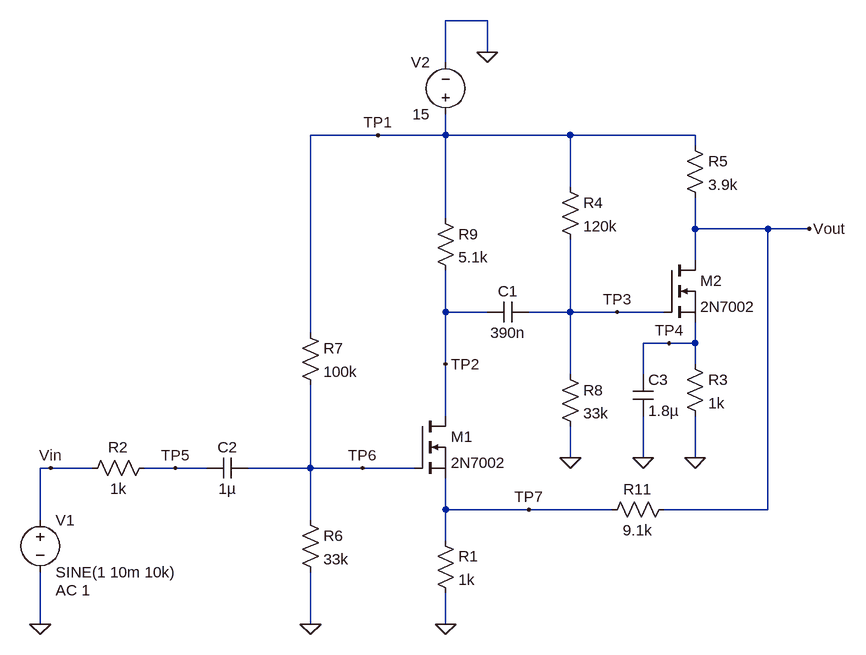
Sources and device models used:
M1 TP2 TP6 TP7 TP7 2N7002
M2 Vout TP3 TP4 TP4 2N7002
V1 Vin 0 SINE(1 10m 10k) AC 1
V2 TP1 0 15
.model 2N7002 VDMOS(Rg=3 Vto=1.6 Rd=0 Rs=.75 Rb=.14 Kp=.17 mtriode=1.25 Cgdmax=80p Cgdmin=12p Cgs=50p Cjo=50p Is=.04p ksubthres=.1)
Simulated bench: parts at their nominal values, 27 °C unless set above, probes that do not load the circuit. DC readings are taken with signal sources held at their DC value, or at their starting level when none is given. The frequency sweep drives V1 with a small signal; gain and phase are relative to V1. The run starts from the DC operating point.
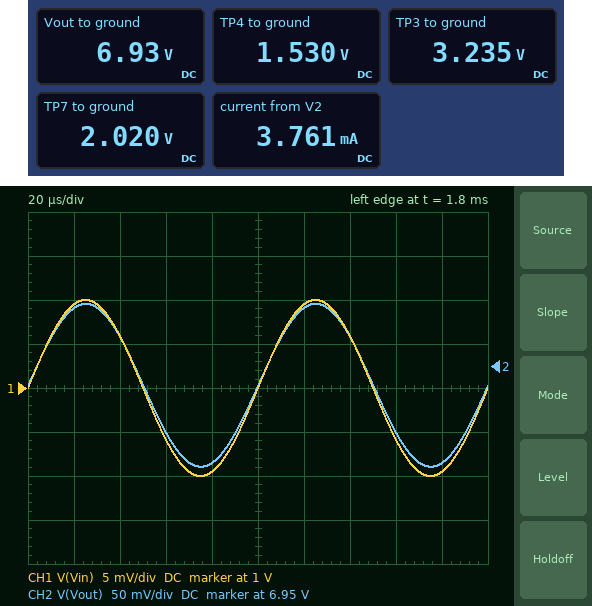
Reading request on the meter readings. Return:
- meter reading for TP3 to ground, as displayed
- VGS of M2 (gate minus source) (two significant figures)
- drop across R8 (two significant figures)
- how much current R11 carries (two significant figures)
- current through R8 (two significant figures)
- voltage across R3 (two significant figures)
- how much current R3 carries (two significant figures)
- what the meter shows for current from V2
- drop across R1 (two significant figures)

3.235 V
1.7 V
3.2 V
540 µA
98 µA
1.5 V
1.5 mA
3.761 mA
2.0 V
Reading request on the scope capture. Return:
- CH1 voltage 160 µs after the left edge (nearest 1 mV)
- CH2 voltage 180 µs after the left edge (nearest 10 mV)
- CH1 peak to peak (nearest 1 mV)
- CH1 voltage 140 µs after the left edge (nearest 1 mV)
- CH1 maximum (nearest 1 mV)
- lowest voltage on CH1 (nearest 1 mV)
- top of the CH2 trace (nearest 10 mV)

994 mV
6.84 V
20 mV
1.006 V
1.010 V
990 mV
7.02 V
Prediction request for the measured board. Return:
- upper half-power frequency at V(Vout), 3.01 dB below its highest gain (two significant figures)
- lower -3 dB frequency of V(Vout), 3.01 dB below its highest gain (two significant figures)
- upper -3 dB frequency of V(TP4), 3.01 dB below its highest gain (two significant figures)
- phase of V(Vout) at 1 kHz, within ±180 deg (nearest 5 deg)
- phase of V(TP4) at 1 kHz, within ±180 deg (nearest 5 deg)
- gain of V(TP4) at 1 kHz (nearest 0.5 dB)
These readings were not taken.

860 kHz
86 Hz
170 Hz
5 deg
100 deg
-11.0 dB
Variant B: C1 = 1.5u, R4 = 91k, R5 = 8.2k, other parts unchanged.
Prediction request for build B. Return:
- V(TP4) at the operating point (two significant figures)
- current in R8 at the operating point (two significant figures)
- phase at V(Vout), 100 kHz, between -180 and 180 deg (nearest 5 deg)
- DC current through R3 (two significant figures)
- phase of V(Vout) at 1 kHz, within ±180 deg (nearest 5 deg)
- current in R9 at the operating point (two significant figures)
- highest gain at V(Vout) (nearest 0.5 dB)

1.7 V
120 µA
-30 deg
1.7 mA
-5 deg
2.0 mA
-18.0 dB
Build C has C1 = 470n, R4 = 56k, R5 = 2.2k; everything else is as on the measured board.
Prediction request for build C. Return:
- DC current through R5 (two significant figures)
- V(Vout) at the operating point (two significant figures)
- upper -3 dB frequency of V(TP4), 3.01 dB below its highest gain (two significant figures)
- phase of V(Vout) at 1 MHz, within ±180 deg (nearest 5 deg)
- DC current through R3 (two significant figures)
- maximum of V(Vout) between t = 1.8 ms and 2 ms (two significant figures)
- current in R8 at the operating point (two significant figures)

4.2 mA
5.8 V
210 Hz
-90 deg
3.8 mA
5.9 V
170 µA
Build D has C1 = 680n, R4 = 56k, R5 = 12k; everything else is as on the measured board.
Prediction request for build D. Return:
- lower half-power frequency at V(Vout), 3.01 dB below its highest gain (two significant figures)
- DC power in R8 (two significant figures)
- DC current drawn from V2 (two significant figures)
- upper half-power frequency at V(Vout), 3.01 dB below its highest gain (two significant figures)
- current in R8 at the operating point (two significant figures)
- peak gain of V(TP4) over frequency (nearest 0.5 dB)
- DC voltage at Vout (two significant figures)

5.7 Hz
940 µW
3.5 mA
120 Hz
170 µA
-22.0 dB
1.2 V
